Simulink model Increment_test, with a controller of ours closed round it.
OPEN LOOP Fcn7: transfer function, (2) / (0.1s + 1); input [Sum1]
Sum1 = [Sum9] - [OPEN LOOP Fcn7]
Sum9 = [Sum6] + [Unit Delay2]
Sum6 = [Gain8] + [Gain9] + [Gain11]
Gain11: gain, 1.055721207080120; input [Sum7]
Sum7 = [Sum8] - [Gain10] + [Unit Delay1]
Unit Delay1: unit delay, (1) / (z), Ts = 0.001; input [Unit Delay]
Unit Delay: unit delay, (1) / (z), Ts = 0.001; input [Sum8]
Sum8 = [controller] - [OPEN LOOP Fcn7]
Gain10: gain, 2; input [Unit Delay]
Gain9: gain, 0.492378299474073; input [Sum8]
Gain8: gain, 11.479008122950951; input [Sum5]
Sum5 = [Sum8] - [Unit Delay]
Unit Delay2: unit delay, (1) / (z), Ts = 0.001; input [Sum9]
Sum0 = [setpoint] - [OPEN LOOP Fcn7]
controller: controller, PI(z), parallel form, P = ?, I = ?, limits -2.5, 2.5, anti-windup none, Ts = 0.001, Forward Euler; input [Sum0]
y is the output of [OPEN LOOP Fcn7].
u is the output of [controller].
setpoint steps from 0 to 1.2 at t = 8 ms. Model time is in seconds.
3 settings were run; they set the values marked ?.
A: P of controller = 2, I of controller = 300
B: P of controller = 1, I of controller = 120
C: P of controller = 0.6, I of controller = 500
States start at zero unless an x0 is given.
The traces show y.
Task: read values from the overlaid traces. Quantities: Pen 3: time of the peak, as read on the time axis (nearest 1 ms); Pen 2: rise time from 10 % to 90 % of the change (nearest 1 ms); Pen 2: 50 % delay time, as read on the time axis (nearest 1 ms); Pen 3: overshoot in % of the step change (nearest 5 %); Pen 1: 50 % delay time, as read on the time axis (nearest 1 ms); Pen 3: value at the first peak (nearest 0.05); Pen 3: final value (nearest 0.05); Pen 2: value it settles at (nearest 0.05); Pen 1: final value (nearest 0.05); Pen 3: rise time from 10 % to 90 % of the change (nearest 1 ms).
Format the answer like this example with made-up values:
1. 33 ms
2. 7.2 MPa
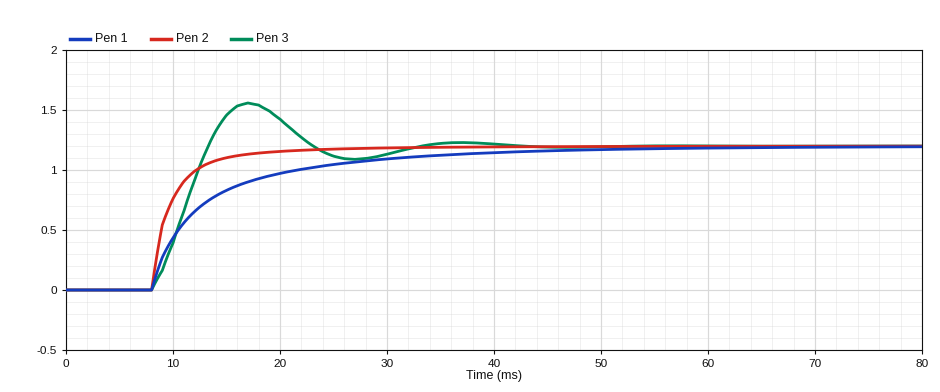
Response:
1. 17 ms
2. 6 ms
3. 9 ms
4. 30 %
5. 11 ms
6. 1.55
7. 1.20
8. 1.20
9. 1.20
10. 4 ms
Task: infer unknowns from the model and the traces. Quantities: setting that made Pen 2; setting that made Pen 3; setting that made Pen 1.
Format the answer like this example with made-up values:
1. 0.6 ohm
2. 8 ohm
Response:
1. A
2. C
3. B
